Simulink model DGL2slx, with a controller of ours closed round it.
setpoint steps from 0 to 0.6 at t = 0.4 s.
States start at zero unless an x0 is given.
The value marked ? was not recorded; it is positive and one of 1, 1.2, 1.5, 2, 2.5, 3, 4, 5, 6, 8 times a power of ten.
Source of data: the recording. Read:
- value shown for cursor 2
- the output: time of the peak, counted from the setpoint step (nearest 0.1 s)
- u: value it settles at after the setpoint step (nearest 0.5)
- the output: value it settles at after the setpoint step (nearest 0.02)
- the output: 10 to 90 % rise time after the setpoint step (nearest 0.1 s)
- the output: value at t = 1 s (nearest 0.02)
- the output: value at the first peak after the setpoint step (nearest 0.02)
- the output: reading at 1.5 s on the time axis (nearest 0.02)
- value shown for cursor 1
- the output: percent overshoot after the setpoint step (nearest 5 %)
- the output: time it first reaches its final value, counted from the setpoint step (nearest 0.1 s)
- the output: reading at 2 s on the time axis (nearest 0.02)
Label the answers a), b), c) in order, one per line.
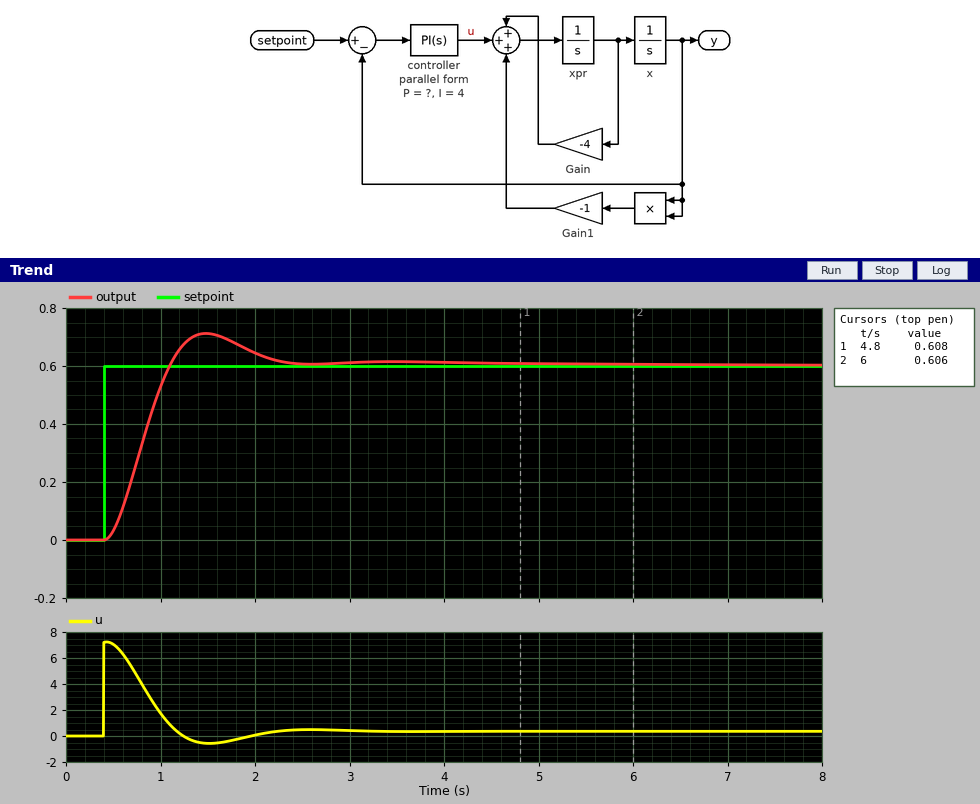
a) 0.606
b) 1.1 s
c) 0.5
d) 0.60
e) 0.5 s
f) 0.52
g) 0.72
h) 0.72
i) 0.608
j) 20 %
k) 0.7 s
l) 0.64
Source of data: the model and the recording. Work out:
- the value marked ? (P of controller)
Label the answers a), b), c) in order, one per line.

a) 12
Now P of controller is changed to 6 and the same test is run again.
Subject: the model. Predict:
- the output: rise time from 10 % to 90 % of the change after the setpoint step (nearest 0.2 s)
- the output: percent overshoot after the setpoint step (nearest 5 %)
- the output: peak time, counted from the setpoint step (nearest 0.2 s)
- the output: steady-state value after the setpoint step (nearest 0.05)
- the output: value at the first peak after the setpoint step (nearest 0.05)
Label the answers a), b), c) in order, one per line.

a) 0.8 s
b) 25 %
c) 1.8 s
d) 0.60
e) 0.75
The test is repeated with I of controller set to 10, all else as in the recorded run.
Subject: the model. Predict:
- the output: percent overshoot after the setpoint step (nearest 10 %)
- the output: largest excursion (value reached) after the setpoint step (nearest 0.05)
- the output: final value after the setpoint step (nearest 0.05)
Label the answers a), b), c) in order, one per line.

a) 30 %
b) 0.80
c) 0.60
